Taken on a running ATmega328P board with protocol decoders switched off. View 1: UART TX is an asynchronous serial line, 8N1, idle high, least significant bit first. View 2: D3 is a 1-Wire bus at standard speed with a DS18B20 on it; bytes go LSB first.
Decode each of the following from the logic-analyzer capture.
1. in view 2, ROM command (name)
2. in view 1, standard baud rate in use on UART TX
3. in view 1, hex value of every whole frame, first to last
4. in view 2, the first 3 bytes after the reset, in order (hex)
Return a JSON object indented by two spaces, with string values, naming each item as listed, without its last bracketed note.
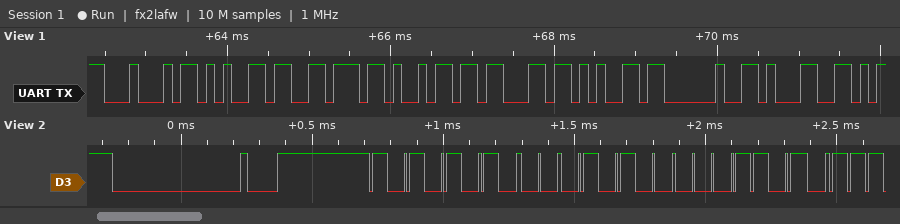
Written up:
{
  "in view 2, ROM command": "Match ROM",
  "in view 1, standard baud rate in use on UART TX": "9600 baud",
  "in view 1, hex value of every whole frame, first to last": "44 65 76 69 63 65 20 31",
  "in view 2, the first 3 bytes after the reset, in order": "55 28 58"
}
